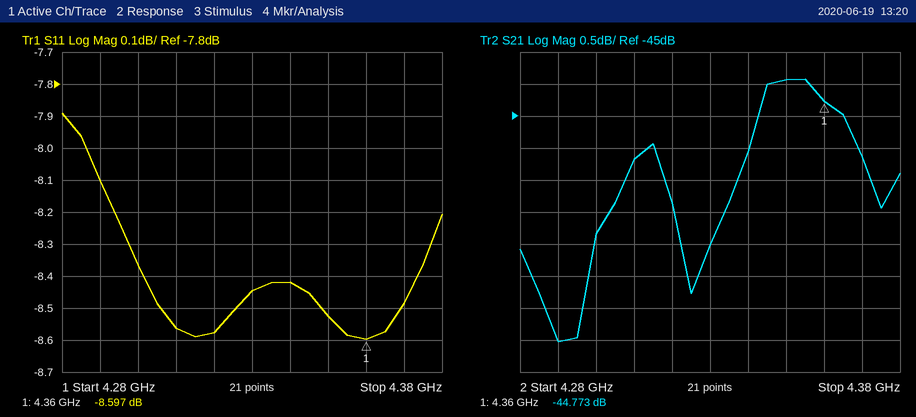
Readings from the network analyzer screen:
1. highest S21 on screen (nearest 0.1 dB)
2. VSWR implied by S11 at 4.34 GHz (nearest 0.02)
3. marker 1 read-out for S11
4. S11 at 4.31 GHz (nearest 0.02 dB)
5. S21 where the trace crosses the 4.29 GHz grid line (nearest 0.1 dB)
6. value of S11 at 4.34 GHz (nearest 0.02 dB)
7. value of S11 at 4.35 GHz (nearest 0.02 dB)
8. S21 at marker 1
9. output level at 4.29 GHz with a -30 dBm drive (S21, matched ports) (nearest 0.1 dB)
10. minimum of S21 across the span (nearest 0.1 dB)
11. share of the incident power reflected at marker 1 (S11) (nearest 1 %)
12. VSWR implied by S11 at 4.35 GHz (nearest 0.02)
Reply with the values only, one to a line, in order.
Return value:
-44.4 dB
2.22
-8.597 dB
-8.56 dB
-48.5 dB
-8.42 dB
-8.52 dB
-44.773 dB
-78.5 dBm
-48.5 dB
14 %
2.20
